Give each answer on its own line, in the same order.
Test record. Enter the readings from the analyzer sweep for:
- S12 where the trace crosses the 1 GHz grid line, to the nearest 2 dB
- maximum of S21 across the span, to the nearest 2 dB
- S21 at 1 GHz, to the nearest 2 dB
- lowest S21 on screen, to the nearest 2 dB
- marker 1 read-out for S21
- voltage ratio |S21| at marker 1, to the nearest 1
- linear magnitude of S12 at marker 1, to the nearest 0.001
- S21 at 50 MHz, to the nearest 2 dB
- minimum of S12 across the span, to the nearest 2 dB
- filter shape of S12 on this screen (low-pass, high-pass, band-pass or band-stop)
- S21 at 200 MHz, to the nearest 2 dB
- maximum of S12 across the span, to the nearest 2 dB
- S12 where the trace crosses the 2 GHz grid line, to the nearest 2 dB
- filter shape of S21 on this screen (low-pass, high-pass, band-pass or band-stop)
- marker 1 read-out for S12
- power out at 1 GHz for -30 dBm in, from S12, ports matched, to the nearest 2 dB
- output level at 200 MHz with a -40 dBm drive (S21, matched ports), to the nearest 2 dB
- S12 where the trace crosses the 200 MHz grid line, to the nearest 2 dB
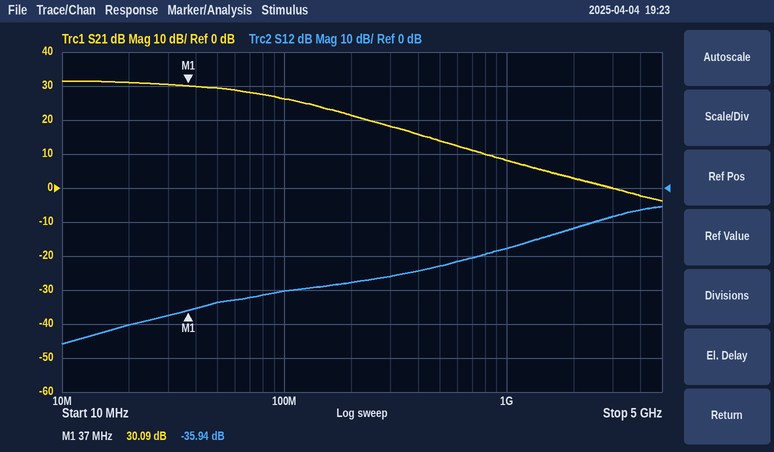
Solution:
-18 dB
32 dB
8 dB
-4 dB
30.09 dB
32
0.016
30 dB
-46 dB
high-pass
22 dB
-6 dB
-12 dB
low-pass
-35.94 dB
-48 dBm
-18 dBm
-28 dB
